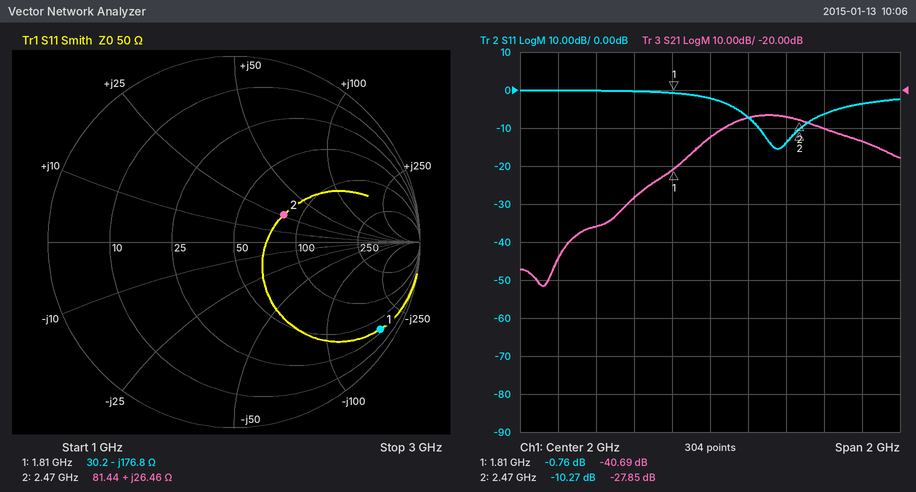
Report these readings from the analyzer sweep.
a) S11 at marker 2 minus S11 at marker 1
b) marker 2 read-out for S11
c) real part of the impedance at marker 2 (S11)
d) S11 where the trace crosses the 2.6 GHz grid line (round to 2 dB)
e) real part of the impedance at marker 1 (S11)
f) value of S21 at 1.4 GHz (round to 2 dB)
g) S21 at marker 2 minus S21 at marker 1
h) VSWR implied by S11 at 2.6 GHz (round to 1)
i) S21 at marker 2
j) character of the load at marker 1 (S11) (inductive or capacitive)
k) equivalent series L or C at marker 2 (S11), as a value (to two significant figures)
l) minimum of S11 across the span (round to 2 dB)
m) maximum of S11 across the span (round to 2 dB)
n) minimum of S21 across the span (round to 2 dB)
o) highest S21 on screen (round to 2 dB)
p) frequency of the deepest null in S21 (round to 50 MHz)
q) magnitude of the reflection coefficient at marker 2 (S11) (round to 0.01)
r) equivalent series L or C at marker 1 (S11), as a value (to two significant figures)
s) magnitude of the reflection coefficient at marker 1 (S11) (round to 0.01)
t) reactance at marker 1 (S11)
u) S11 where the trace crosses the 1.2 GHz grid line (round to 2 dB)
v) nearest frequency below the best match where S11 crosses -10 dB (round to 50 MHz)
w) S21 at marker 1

-9.51 dB
-10.27 dB
81.44 Ω
-6 dB
30.2 Ω
-56 dB
12.84 dB
3
-27.85 dB
capacitive
1.7 nH
-16 dB
0 dB
-72 dB
-26 dB
1.10 GHz
0.31
500 fF
0.92
-176.8 Ω
0 dB
2.25 GHz
-40.69 dB
